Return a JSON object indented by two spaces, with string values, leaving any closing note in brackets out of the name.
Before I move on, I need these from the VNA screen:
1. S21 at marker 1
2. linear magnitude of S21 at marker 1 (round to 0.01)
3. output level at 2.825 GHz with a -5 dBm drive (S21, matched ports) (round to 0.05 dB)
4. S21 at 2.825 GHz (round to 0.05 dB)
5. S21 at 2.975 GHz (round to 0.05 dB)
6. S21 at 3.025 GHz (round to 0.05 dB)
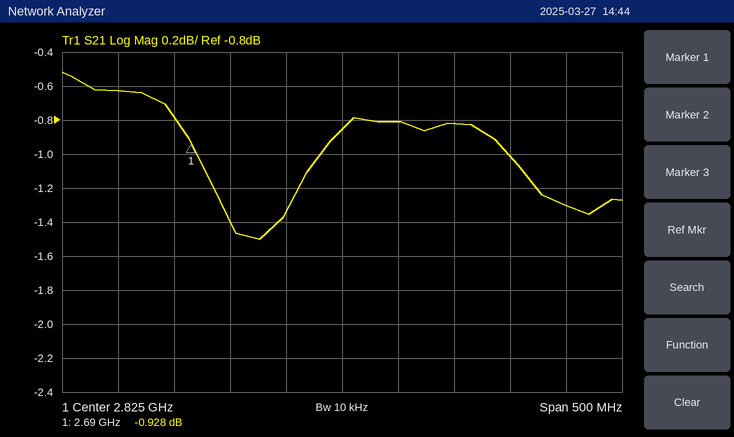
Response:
{
  "S21 at marker 1": "-0.928 dB",
  "linear magnitude of S21 at marker 1": "0.90",
  "output level at 2.825 GHz with a -5 dBm drive (S21, matched ports)": "-5.85 dBm",
  "S21 at 2.825 GHz": "-0.85 dB",
  "S21 at 2.975 GHz": "-1.00 dB",
  "S21 at 3.025 GHz": "-1.30 dB"
}
